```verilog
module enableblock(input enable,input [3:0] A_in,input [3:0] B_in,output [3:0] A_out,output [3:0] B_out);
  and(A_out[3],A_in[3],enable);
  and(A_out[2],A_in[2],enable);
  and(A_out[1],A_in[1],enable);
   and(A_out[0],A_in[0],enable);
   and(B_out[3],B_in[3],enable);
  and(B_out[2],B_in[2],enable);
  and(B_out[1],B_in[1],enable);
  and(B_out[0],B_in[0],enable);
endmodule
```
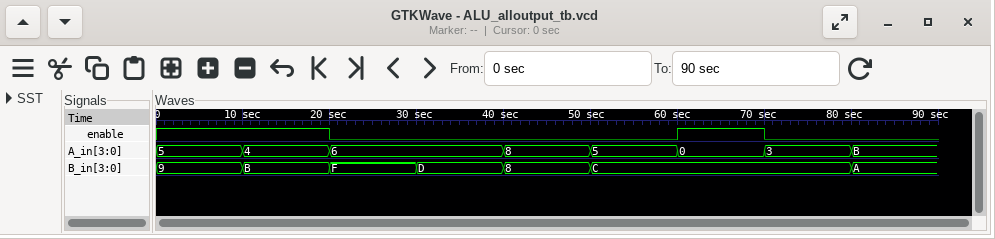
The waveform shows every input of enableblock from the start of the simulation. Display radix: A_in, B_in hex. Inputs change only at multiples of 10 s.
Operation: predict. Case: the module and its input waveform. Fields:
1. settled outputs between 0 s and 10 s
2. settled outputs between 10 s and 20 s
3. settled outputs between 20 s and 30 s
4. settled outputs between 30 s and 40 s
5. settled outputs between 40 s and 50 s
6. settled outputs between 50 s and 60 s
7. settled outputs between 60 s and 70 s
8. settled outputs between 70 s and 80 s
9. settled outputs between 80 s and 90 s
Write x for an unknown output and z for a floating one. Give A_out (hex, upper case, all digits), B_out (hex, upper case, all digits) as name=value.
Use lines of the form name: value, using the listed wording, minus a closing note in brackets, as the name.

settled outputs between 0 s and 10 s: A_out=5, B_out=9
settled outputs between 10 s and 20 s: A_out=4, B_out=B
settled outputs between 20 s and 30 s: A_out=0, B_out=0
settled outputs between 30 s and 40 s: A_out=0, B_out=0
settled outputs between 40 s and 50 s: A_out=0, B_out=0
settled outputs between 50 s and 60 s: A_out=0, B_out=0
settled outputs between 60 s and 70 s: A_out=0, B_out=C
settled outputs between 70 s and 80 s: A_out=0, B_out=0
settled outputs between 80 s and 90 s: A_out=0, B_out=0
